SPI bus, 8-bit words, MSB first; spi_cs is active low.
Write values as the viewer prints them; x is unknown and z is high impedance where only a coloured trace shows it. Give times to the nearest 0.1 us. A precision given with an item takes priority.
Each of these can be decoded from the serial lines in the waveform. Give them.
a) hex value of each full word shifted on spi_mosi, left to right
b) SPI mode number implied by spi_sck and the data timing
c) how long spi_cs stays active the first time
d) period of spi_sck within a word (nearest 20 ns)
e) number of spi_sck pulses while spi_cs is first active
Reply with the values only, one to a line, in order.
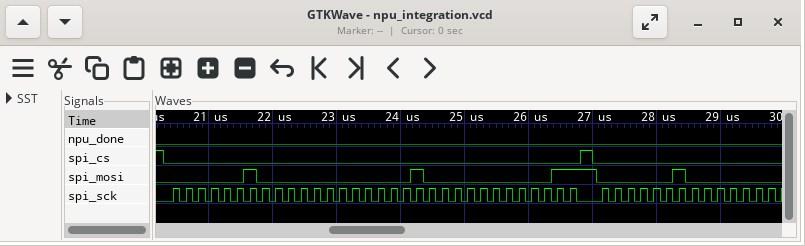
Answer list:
02, 00, 10, 03, 02
0
6.5 us
200 ns
32
